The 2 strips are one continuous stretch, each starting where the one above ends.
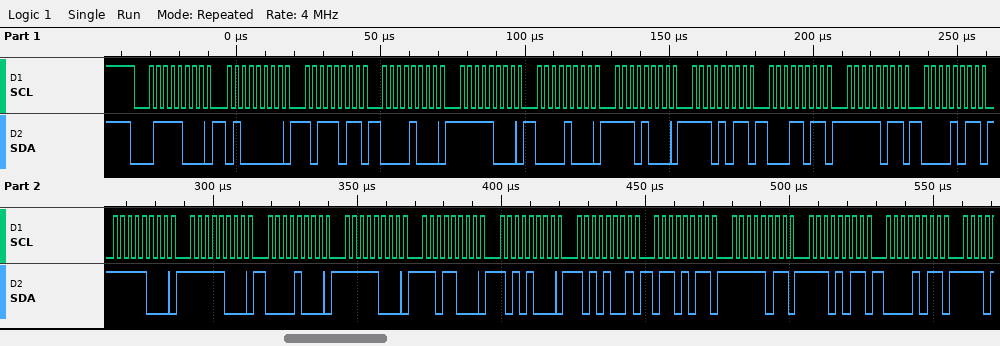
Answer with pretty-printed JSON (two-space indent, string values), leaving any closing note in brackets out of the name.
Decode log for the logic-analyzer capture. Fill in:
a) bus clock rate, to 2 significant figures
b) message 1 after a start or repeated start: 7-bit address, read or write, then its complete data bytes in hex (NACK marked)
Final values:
{
  "bus clock rate, to 2 significant figures": "400 kHz",
  "message 1 after a start or repeated start: 7-bit address, read or write, then its complete data bytes in hex": "0x3C write: 40 BB 08 F8 08 E8 EB 1B FB 0B F8 F8 08 F8 D8 A8 A9 6B FB EB 0B"
}
